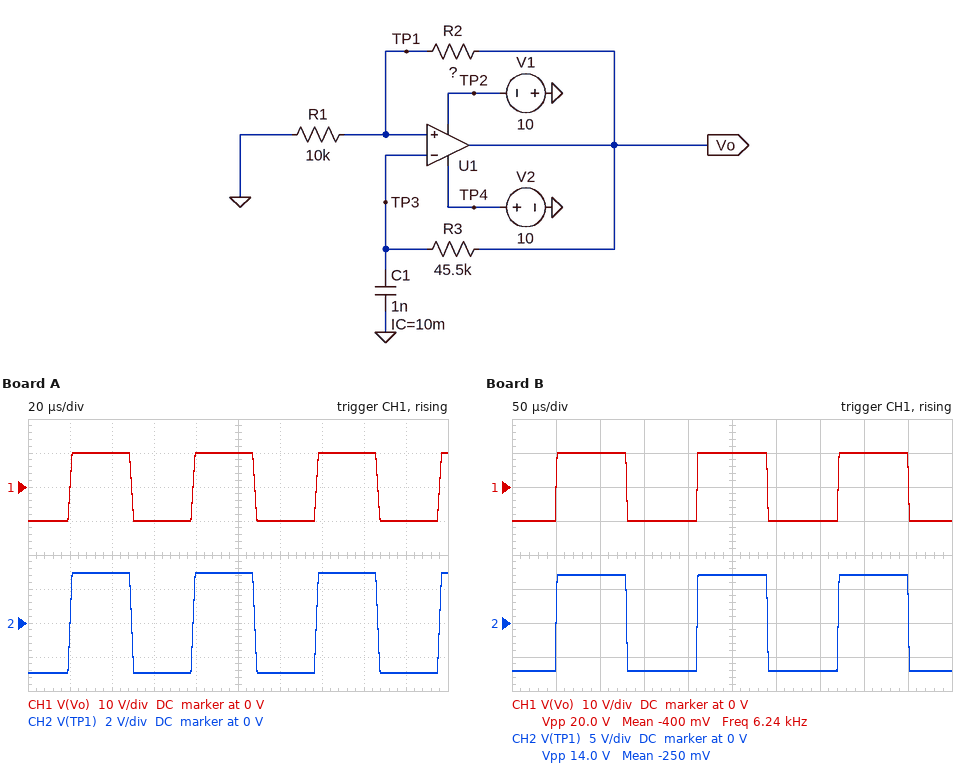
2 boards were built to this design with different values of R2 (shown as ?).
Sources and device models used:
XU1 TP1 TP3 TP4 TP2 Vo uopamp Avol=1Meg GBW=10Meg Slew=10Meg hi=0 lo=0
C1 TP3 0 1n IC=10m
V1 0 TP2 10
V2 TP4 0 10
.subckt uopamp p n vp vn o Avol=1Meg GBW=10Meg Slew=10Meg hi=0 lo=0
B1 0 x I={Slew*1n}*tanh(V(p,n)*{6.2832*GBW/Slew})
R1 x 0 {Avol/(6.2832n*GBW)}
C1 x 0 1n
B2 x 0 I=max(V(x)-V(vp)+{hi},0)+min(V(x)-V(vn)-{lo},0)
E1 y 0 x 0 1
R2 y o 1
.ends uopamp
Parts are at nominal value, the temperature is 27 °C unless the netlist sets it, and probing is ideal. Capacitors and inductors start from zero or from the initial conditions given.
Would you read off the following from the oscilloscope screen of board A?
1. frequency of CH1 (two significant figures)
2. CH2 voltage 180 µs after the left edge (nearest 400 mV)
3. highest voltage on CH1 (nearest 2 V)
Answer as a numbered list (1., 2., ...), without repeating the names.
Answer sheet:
1. 17 kHz
2. -2.8 V
3. 10 V
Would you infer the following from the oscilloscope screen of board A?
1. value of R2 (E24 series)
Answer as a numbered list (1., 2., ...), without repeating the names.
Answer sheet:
1. 24 kΩ
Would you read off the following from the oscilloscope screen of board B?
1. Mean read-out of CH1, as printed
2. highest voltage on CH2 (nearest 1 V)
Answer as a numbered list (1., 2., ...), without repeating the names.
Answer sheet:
1. -400 mV
2. 7 V
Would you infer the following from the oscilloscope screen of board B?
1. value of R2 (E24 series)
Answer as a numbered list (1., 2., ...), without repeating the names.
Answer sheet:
1. 4.3 kΩ
